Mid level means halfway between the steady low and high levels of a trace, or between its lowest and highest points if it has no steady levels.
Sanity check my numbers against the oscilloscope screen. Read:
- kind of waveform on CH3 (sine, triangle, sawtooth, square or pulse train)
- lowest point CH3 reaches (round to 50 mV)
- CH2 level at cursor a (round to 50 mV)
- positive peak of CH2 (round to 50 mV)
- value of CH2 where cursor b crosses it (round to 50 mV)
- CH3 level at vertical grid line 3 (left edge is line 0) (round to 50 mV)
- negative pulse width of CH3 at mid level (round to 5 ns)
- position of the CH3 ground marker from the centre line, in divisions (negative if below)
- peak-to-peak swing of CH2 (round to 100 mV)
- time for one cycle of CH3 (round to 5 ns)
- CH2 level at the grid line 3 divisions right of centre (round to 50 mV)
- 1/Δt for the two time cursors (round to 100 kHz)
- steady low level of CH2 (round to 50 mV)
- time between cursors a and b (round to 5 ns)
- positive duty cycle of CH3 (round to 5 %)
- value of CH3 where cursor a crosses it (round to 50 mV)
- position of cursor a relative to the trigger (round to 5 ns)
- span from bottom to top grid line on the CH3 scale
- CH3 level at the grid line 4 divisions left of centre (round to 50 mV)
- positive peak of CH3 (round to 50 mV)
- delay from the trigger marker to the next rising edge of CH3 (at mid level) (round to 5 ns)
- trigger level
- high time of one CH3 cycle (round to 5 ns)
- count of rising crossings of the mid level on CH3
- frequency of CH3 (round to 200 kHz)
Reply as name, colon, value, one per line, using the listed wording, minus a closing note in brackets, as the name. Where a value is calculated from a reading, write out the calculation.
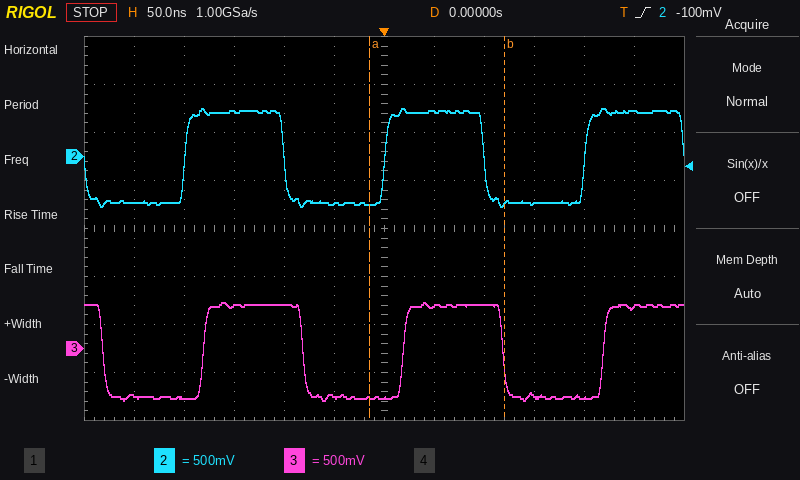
kind of waveform on CH3: square
lowest point CH3 reaches: -550 mV
CH2 level at cursor a: -500 mV
positive peak of CH2: 500 mV
value of CH2 where cursor b crosses it: -500 mV
CH3 level at vertical grid line 3 (left edge is line 0): 450 mV
negative pulse width of CH3 at mid level: 100 ns
position of the CH3 ground marker from the centre line, in divisions: -2.5 div
peak-to-peak swing of CH2: 1.00 V
time for one cycle of CH3: 200 ns
CH2 level at the grid line 3 divisions right of centre: -500 mV
1/Δt for the two time cursors: 1 / 135 ns ≈ 7.4 MHz
steady low level of CH2: -500 mV
time between cursors a and b: 135 ns
positive duty cycle of CH3: 100 ns / 200 ns ≈ 50 %
value of CH3 where cursor a crosses it: -500 mV
position of cursor a relative to the trigger: -15 ns
span from bottom to top grid line on the CH3 scale: 4 V
CH3 level at the grid line 4 divisions left of centre: -500 mV
positive peak of CH3: 500 mV
delay from the trigger marker to the next rising edge of CH3 (at mid level): 20 ns
trigger level: -100 mV
high time of one CH3 cycle: 100 ns
count of rising crossings of the mid level on CH3: 3
frequency of CH3: 1 / 200 ns ≈ 5.0 MHz
